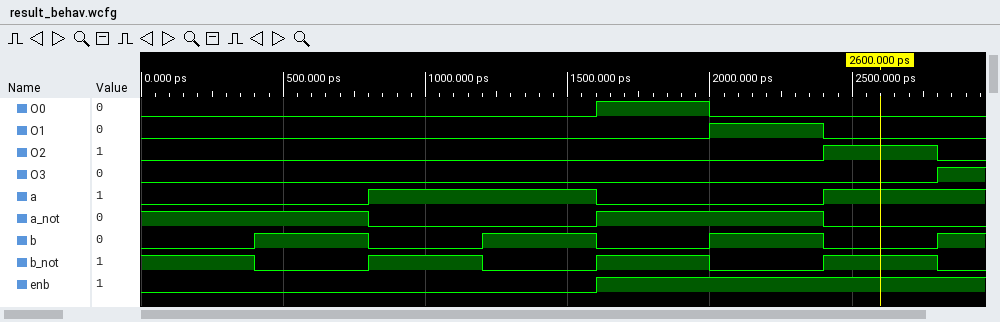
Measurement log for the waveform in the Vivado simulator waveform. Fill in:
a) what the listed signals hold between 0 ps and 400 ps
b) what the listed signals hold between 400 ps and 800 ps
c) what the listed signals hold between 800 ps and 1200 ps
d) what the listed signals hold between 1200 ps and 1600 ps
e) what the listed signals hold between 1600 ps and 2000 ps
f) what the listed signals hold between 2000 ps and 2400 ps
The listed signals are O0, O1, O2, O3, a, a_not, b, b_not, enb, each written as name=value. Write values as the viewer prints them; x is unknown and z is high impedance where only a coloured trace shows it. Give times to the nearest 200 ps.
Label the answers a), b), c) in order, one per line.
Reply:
a) O0=0, O1=0, O2=0, O3=0, a=0, a_not=1, b=0, b_not=1, enb=0
b) O0=0, O1=0, O2=0, O3=0, a=0, a_not=1, b=1, b_not=0, enb=0
c) O0=0, O1=0, O2=0, O3=0, a=1, a_not=0, b=0, b_not=1, enb=0
d) O0=0, O1=0, O2=0, O3=0, a=1, a_not=0, b=1, b_not=0, enb=0
e) O0=1, O1=0, O2=0, O3=0, a=0, a_not=1, b=0, b_not=1, enb=1
f) O0=0, O1=1, O2=0, O3=0, a=0, a_not=1, b=1, b_not=0, enb=1
